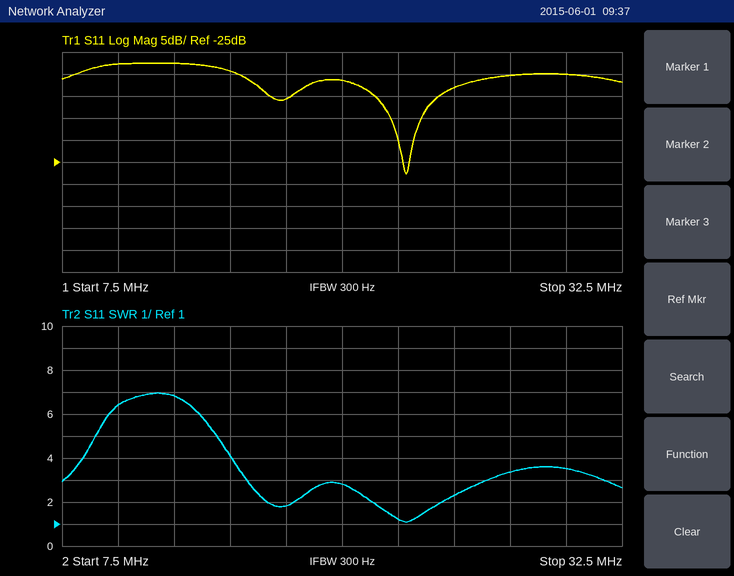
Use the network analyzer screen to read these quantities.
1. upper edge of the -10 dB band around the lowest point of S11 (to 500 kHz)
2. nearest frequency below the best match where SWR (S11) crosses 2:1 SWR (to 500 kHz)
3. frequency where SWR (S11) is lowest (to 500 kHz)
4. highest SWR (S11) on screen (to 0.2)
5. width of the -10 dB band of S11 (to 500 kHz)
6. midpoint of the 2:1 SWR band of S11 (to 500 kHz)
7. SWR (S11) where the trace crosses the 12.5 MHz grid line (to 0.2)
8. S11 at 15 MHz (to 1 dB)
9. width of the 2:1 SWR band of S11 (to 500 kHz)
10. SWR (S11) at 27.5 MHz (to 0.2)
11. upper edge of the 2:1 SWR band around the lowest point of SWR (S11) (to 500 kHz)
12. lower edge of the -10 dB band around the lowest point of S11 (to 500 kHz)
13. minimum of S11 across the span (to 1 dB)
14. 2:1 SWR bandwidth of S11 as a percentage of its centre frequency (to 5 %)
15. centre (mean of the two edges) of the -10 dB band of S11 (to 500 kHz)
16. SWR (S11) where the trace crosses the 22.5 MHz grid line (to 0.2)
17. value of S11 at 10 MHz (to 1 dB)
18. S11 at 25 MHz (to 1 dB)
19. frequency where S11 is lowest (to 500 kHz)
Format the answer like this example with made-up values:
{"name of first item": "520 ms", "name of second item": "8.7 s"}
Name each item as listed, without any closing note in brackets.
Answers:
{"upper edge of the -10 dB band around the lowest point of S11": "24.5 MHz", "nearest frequency below the best match where SWR (S11) crosses 2:1 SWR": "21.5 MHz", "frequency where SWR (S11) is lowest": "23.0 MHz", "highest SWR (S11) on screen": "7.0", "width of the -10 dB band of S11": "3.0 MHz", "midpoint of the 2:1 SWR band of S11": "23.0 MHz", "SWR (S11) where the trace crosses the 12.5 MHz grid line": "6.8", "S11 at 15 MHz": "-4 dB", "width of the 2:1 SWR band of S11": "3.0 MHz", "SWR (S11) at 27.5 MHz": "3.4", "upper edge of the 2:1 SWR band around the lowest point of SWR (S11)": "24.5 MHz", "lower edge of the -10 dB band around the lowest point of S11": "21.5 MHz", "minimum of S11 across the span": "-28 dB", "2:1 SWR bandwidth of S11 as a percentage of its centre frequency": "15 %", "centre (mean of the two edges) of the -10 dB band of S11": "23.0 MHz", "SWR (S11) where the trace crosses the 22.5 MHz grid line": "1.2", "value of S11 at 10 MHz": "-3 dB", "S11 at 25 MHz": "-8 dB", "frequency where S11 is lowest": "23.0 MHz"}
